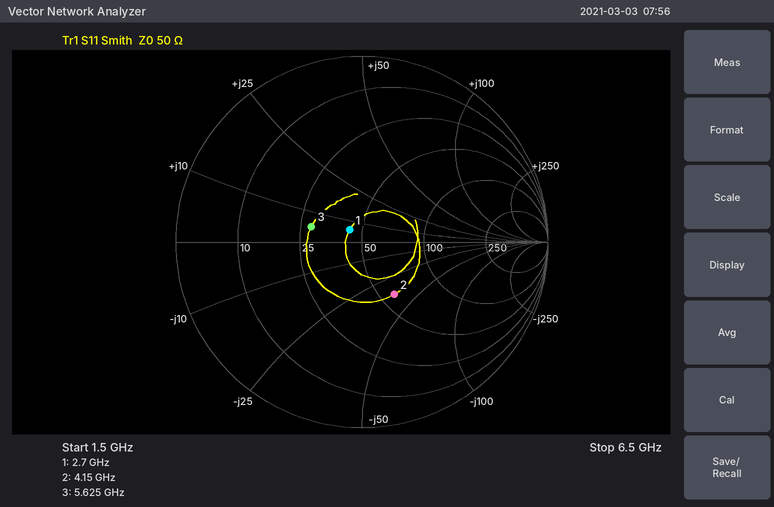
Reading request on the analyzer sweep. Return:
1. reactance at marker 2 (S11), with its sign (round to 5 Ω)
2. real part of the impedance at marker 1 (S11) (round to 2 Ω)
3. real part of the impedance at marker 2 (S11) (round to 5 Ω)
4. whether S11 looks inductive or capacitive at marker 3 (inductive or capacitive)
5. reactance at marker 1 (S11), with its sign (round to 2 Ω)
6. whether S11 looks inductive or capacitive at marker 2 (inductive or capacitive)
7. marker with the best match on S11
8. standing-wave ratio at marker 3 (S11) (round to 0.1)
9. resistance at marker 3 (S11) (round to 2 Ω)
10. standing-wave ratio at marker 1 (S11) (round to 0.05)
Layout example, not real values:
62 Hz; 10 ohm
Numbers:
-35 Ω; 44 Ω; 60 Ω; inductive; +6 Ω; capacitive; marker 1; 1.8; 28 Ω; 1.20
